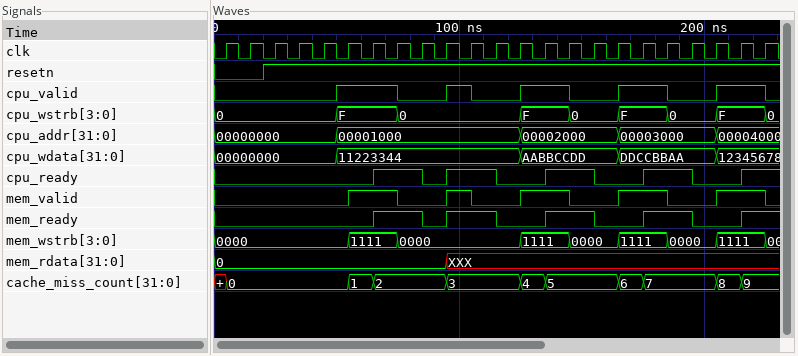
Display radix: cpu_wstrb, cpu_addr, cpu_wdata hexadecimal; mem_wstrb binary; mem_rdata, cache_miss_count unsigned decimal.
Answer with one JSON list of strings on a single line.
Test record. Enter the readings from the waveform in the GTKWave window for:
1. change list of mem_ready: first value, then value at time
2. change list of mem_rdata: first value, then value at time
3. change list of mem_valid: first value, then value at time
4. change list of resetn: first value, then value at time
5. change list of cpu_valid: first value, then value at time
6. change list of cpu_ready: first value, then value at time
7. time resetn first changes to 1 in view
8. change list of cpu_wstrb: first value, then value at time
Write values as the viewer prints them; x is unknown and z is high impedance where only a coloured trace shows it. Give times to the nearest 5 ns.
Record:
["0, 1 at 65 ns, 0 at 85 ns, 1 at 95 ns, 0 at 115 ns, 1 at 135 ns, 0 at 155 ns, 1 at 175 ns, 0 at 195 ns, 1 at 215 ns", "0, XXX at 95 ns", "0, 1 at 55 ns, 0 at 75 ns, 1 at 95 ns, 0 at 105 ns, 1 at 125 ns, 0 at 145 ns, 1 at 165 ns, 0 at 185 ns, 1 at 205 ns, 0 at 225 ns", "0, 1 at 20 ns", "0, 1 at 50 ns, 0 at 75 ns, 1 at 95 ns, 0 at 105 ns, 1 at 125 ns, 0 at 145 ns, 1 at 165 ns, 0 at 185 ns, 1 at 205 ns, 0 at 225 ns", "0, 1 at 65 ns, 0 at 85 ns, 1 at 95 ns, 0 at 115 ns, 1 at 135 ns, 0 at 155 ns, 1 at 175 ns, 0 at 195 ns, 1 at 215 ns", "20 ns", "0, F at 50 ns, 0 at 75 ns, F at 125 ns, 0 at 145 ns, F at 165 ns, 0 at 185 ns, F at 205 ns, 0 at 225 ns"]
